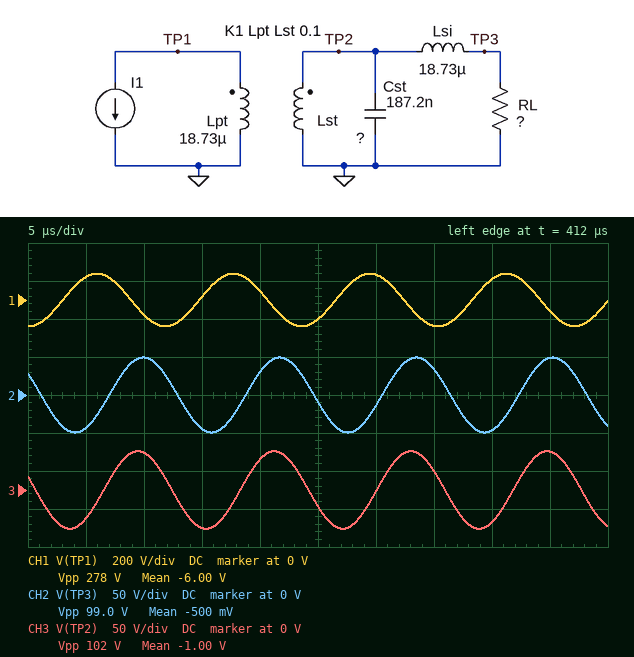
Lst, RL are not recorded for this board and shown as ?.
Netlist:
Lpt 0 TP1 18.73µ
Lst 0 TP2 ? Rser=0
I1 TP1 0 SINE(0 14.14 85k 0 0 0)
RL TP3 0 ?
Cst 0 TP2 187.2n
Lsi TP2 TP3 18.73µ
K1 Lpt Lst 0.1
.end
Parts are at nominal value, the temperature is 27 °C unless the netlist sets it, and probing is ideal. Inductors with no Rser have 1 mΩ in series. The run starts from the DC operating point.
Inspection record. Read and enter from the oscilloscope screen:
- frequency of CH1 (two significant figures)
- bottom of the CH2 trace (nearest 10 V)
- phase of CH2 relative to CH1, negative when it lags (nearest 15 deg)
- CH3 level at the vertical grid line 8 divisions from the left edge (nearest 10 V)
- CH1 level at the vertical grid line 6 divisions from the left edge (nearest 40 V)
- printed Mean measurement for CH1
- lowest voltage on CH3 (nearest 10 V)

85 kHz
-50 V
-120 deg
-40 V
120 V
-6.00 V
-50 V
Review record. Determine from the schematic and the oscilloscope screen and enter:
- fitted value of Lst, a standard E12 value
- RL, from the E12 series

22 µH
39 Ω
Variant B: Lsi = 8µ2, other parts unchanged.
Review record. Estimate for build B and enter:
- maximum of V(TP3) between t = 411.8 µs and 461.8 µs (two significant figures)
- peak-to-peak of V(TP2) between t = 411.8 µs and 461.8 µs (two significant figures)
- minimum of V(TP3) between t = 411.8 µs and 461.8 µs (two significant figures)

46 V
93 V
-46 V
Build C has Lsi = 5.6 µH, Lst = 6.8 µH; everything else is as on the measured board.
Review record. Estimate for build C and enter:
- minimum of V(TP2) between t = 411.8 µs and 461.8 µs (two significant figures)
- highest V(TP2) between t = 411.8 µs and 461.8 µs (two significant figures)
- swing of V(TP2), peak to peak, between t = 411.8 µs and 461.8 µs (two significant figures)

-13 V
13 V
26 V
